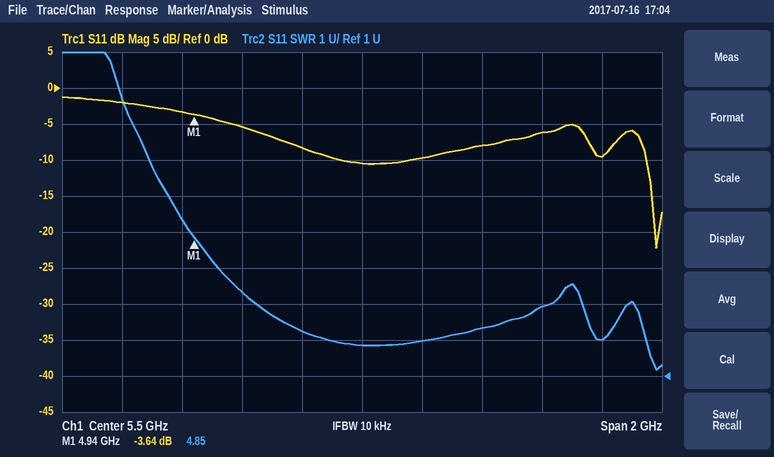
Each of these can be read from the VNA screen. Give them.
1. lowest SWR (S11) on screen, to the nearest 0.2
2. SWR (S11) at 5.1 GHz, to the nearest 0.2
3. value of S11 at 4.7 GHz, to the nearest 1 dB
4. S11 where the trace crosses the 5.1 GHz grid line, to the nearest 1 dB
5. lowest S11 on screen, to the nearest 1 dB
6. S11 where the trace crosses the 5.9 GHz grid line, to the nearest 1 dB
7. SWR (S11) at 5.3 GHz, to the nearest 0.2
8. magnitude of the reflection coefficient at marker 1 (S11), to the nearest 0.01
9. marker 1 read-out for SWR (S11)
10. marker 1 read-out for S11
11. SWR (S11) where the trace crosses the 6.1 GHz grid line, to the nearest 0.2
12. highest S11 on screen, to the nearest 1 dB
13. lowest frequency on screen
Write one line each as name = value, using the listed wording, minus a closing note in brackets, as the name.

lowest SWR (S11) on screen, to the nearest 0.2 = 1.2
SWR (S11) at 5.1 GHz, to the nearest 0.2 = 3.4
value of S11 at 4.7 GHz, to the nearest 1 dB = -2 dB
S11 where the trace crosses the 5.1 GHz grid line, to the nearest 1 dB = -5 dB
lowest S11 on screen, to the nearest 1 dB = -22 dB
S11 where the trace crosses the 5.9 GHz grid line, to the nearest 1 dB = -8 dB
SWR (S11) at 5.3 GHz, to the nearest 0.2 = 2.2
magnitude of the reflection coefficient at marker 1 (S11), to the nearest 0.01 = 0.66
marker 1 read-out for SWR = 4.85
marker 1 read-out for S11 = -3.64 dB
SWR (S11) where the trace crosses the 6.1 GHz grid line, to the nearest 0.2 = 3.0
highest S11 on screen, to the nearest 1 dB = -1 dB
lowest frequency on screen = 4.5 GHz
